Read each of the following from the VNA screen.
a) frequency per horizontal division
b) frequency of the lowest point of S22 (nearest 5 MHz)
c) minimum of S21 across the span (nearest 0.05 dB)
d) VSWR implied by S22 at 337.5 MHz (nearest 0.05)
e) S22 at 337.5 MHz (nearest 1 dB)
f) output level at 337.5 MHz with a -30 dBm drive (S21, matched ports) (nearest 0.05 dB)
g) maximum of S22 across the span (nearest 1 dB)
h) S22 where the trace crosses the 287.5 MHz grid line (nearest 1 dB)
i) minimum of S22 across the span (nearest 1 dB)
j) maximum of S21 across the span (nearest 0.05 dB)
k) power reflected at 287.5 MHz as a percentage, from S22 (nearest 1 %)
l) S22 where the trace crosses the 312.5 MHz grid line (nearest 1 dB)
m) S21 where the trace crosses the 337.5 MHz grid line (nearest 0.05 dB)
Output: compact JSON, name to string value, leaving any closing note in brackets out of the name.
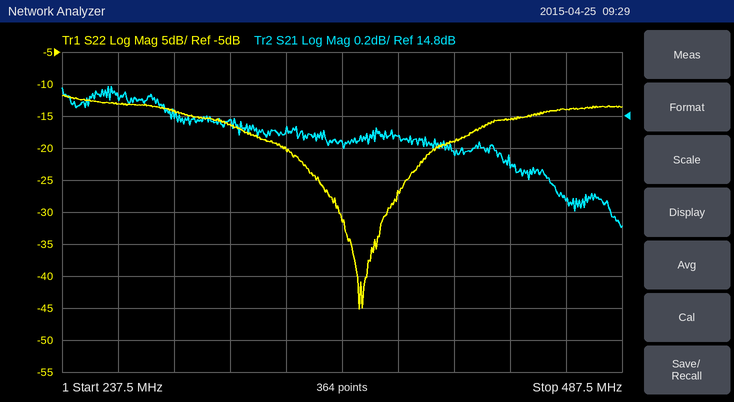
{"frequency per horizontal division": "25 MHz", "frequency of the lowest point of S22": "370 MHz", "minimum of S21 across the span": "14.10 dB", "VSWR implied by S22 at 337.5 MHz": "1.20", "S22 at 337.5 MHz": "-20 dB", "output level at 337.5 MHz with a -30 dBm drive (S21, matched ports)": "-15.30 dBm", "maximum of S22 across the span": "-12 dB", "S22 where the trace crosses the 287.5 MHz grid line": "-14 dB", "minimum of S22 across the span": "-45 dB", "maximum of S21 across the span": "15.00 dB", "power reflected at 287.5 MHz as a percentage, from S22": "4 %", "S22 where the trace crosses the 312.5 MHz grid line": "-16 dB", "S21 where the trace crosses the 337.5 MHz grid line": "14.70 dB"}
